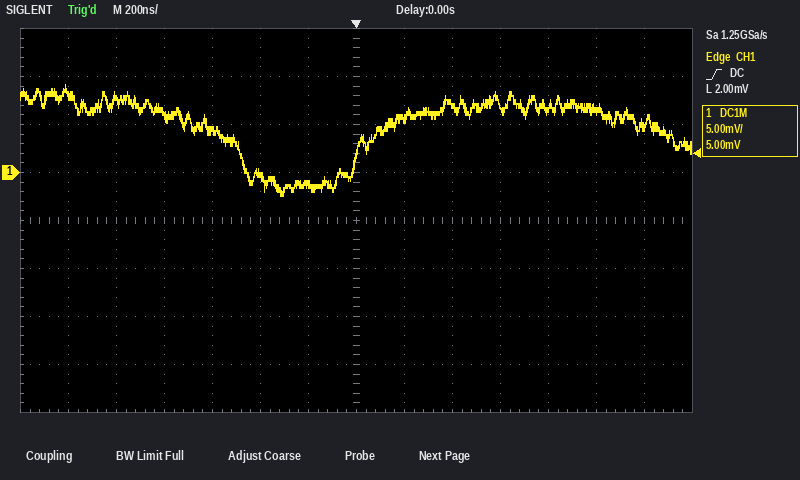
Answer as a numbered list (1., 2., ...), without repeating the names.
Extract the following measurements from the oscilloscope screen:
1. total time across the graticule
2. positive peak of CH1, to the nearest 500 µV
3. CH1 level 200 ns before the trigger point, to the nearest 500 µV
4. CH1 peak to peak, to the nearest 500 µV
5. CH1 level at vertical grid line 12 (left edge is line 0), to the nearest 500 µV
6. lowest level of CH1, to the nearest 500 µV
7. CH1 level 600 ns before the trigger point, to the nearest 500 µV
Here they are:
1. 2.8 µs
2. 9.0 mV
3. -1.0 mV
4. 11.5 mV
5. 6.5 mV
6. -2.5 mV
7. 4.5 mV
